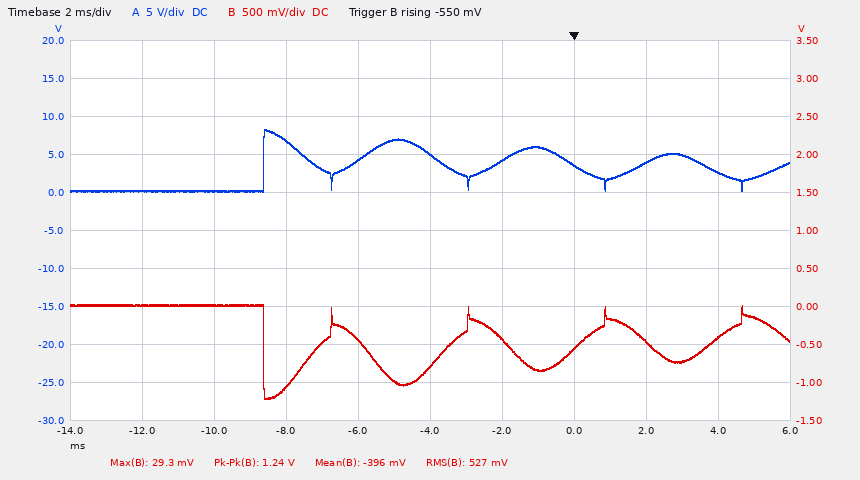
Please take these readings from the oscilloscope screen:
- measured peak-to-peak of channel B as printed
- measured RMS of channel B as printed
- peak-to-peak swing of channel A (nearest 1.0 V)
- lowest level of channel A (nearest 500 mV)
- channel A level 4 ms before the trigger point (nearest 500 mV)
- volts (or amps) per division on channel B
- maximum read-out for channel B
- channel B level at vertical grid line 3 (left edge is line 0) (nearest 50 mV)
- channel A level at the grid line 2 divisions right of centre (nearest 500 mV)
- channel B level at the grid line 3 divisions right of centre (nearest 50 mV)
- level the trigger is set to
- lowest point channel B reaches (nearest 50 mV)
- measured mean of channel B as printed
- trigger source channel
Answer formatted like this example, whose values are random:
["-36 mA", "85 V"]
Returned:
["1.24 V", "527 mV", "8.0 V", "0.0 V", "5.0 V", "500 mV", "29.3 mV", "-1.05 V", "3.5 V", "-450 mV", "-550 mV", "-1.20 V", "-396 mV", "channel B"]
